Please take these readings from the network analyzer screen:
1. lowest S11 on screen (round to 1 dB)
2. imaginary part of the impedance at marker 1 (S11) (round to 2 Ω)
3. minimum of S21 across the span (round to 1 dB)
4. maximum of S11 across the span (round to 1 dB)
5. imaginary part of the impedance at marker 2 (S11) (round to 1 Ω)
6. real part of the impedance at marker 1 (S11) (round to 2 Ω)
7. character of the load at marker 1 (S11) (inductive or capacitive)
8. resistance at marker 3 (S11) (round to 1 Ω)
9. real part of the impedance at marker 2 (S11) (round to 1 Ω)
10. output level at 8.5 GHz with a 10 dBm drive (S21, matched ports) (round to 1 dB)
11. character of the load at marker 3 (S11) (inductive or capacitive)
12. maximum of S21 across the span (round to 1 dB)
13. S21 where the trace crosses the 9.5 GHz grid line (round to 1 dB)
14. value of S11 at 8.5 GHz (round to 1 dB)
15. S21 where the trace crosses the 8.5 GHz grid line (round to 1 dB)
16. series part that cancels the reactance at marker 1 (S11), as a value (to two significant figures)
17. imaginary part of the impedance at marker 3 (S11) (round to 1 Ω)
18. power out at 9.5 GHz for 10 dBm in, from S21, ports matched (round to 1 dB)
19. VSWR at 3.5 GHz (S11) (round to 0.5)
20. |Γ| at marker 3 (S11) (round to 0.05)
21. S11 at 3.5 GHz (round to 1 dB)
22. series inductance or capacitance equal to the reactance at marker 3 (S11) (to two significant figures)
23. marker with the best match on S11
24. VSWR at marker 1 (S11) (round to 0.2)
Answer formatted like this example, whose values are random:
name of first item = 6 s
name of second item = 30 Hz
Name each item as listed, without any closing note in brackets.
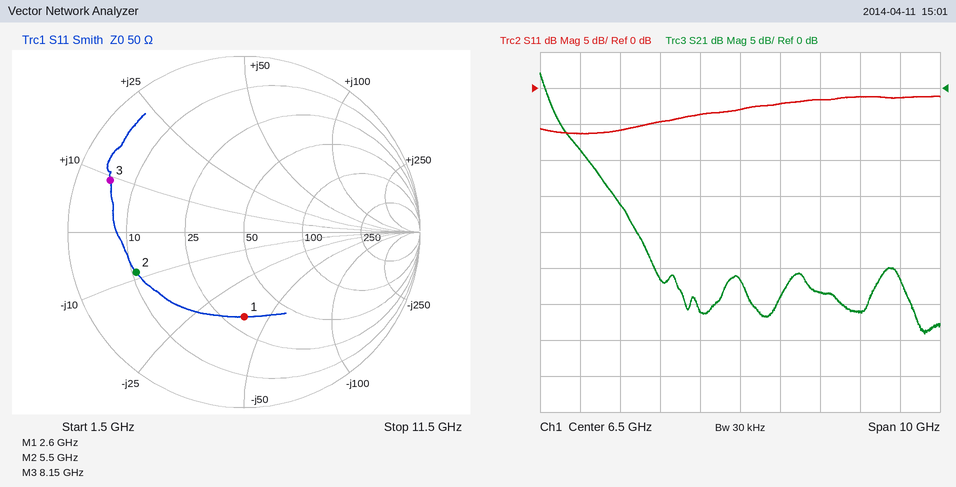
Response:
lowest S11 on screen = -6 dB
imaginary part of the impedance at marker 1 (S11) = -40 Ω
minimum of S21 across the span = -34 dB
maximum of S11 across the span = -1 dB
imaginary part of the impedance at marker 2 (S11) = -9 Ω
real part of the impedance at marker 1 (S11) = 32 Ω
character of the load at marker 1 (S11) = capacitive
resistance at marker 3 (S11) = 5 Ω
real part of the impedance at marker 2 (S11) = 11 Ω
output level at 8.5 GHz with a 10 dBm drive (S21, matched ports) = -18 dBm
character of the load at marker 3 (S11) = inductive
maximum of S21 across the span = 2 dB
S21 where the trace crosses the 9.5 GHz grid line = -31 dB
value of S11 at 8.5 GHz = -2 dB
S21 where the trace crosses the 8.5 GHz grid line = -28 dB
series part that cancels the reactance at marker 1 (S11), as a value = 2.4 nH
imaginary part of the impedance at marker 3 (S11) = +9 Ω
power out at 9.5 GHz for 10 dBm in, from S21, ports matched = -21 dBm
VSWR at 3.5 GHz (S11) = 3.0
|Γ| at marker 3 (S11) = 0.80
S11 at 3.5 GHz = -6 dB
series inductance or capacitance equal to the reactance at marker 3 (S11) = 180 pH
marker with the best match on S11 = marker 1
VSWR at marker 1 (S11) = 2.8
